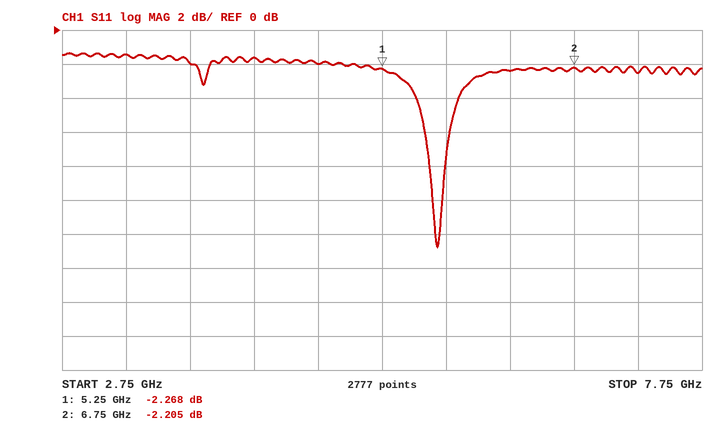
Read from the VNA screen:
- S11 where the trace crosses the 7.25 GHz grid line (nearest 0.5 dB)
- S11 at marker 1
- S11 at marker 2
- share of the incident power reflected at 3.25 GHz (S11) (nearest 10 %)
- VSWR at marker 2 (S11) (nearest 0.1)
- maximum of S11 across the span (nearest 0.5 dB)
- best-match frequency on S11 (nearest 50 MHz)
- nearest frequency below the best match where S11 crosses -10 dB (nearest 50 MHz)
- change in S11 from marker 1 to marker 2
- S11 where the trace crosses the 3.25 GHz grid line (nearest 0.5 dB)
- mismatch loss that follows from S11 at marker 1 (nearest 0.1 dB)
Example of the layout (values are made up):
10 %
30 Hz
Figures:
-2.5 dB
-2.268 dB
-2.205 dB
70 %
7.9
-1.5 dB
5.70 GHz
5.65 GHz
0.063 dB
-1.5 dB
3.9 dB
